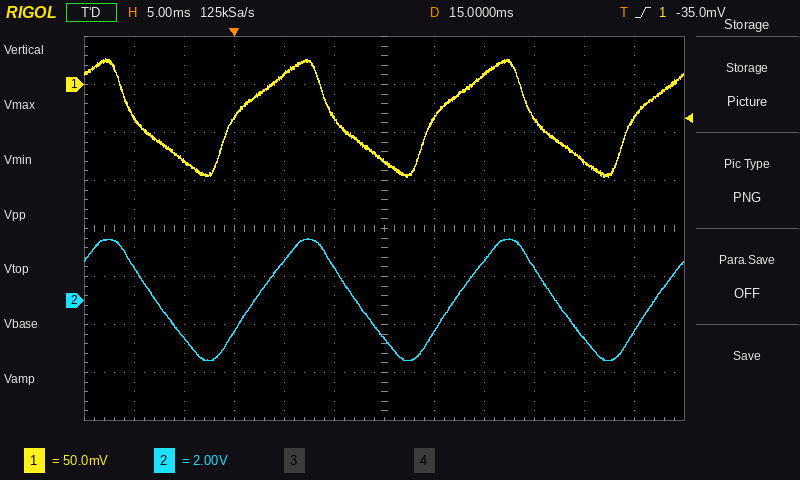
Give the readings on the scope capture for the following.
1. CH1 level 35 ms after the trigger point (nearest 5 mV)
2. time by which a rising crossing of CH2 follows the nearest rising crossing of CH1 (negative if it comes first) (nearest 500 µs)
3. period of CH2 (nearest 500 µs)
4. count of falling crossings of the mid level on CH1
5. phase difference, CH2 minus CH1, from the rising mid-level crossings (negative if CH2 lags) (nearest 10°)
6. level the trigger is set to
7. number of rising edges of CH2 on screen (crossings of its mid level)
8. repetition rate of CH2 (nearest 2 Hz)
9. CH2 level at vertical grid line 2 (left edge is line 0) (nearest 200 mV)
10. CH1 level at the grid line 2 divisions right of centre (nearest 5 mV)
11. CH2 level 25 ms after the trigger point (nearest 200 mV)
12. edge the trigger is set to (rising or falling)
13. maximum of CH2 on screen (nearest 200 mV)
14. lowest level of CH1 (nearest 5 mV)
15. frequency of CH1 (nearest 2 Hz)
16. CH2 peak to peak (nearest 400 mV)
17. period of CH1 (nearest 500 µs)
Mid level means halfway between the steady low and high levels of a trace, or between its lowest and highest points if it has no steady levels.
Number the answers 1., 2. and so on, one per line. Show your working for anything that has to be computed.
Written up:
1. -80 mV
2. +2.0 ms
3. 20.0 ms
4. 3
5. −360° × (+2.0 ms) / 20.0 ms ≈ -36.0°, so -40° to the nearest 10°
6. -35.0 mV
7. 3
8. 1 / 20.0 ms ≈ 50 Hz
9. -1.6 V
10. 10 mV
11. 1.6 V
12. rising
13. 2.6 V
14. -95 mV
15. 1 / 20.0 ms ≈ 50 Hz
16. 5.2 V
17. 20.0 ms
